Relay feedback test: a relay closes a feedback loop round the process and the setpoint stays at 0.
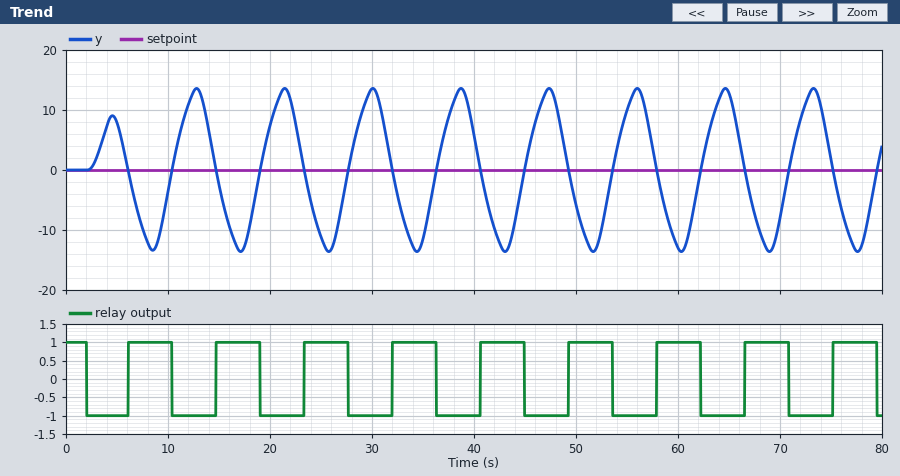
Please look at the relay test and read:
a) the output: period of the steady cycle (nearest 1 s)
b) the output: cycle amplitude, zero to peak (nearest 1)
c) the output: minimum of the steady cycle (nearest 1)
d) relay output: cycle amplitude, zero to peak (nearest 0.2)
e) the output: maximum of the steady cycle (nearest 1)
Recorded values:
9 s
14
-14
1.0
14
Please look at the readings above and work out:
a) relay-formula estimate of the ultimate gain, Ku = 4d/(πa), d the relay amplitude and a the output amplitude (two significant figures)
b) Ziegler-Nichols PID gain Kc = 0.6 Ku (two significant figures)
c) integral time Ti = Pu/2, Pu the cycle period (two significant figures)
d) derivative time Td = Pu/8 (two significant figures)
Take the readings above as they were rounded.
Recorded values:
0.091
0.055
4.5 s
1.1 s
